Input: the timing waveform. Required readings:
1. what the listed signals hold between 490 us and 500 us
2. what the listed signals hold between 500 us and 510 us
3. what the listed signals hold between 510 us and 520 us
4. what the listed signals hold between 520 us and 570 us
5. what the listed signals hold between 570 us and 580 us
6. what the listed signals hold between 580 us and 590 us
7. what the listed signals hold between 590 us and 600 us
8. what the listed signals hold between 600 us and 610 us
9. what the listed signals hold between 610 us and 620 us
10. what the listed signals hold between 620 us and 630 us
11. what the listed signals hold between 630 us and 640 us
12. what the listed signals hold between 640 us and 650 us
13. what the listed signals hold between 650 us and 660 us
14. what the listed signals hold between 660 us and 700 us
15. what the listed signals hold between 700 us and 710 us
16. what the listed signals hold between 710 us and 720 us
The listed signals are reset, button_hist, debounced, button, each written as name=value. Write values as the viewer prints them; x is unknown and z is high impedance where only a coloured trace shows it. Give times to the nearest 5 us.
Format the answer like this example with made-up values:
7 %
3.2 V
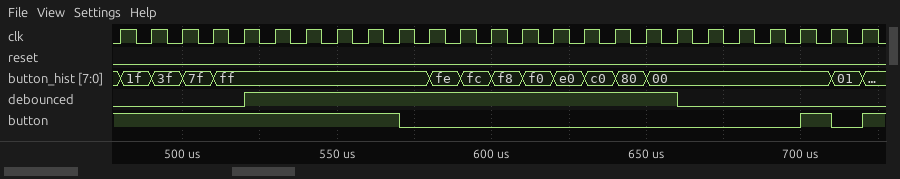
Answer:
reset=0, button_hist=3f, debounced=0, button=1
reset=0, button_hist=7f, debounced=0, button=1
reset=0, button_hist=ff, debounced=0, button=1
reset=0, button_hist=ff, debounced=1, button=1
reset=0, button_hist=ff, debounced=1, button=0
reset=0, button_hist=fe, debounced=1, button=0
reset=0, button_hist=fc, debounced=1, button=0
reset=0, button_hist=f8, debounced=1, button=0
reset=0, button_hist=f0, debounced=1, button=0
reset=0, button_hist=e0, debounced=1, button=0
reset=0, button_hist=c0, debounced=1, button=0
reset=0, button_hist=80, debounced=1, button=0
reset=0, button_hist=00, debounced=1, button=0
reset=0, button_hist=00, debounced=0, button=0
reset=0, button_hist=00, debounced=0, button=1
reset=0, button_hist=01, debounced=0, button=0
